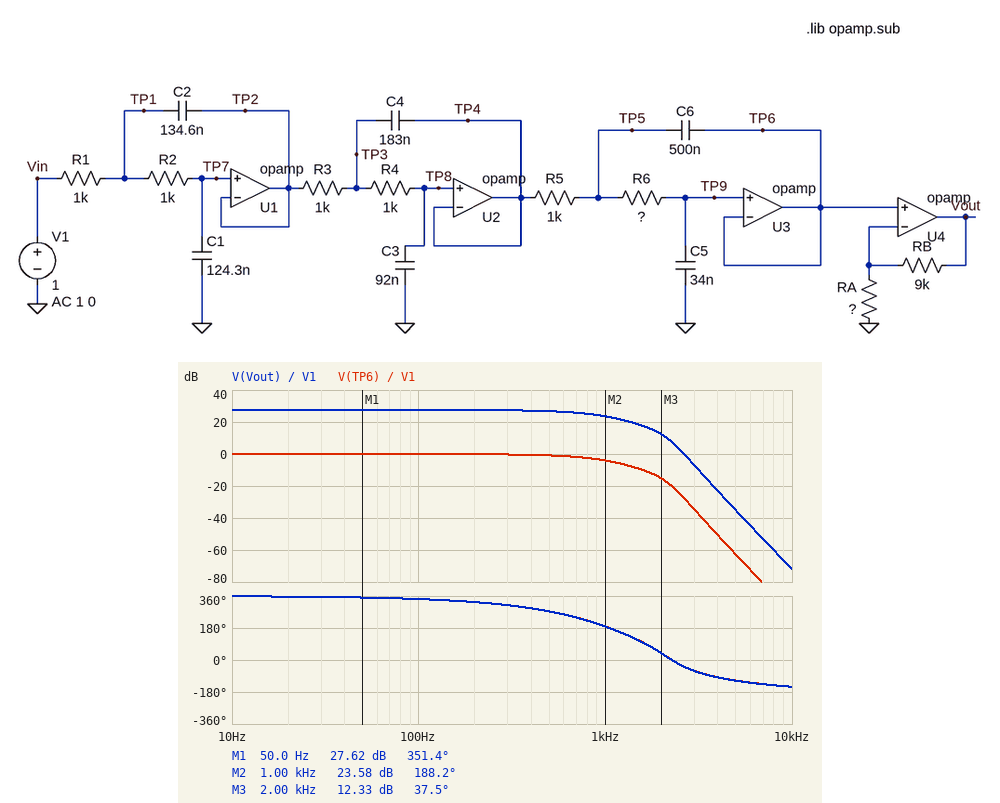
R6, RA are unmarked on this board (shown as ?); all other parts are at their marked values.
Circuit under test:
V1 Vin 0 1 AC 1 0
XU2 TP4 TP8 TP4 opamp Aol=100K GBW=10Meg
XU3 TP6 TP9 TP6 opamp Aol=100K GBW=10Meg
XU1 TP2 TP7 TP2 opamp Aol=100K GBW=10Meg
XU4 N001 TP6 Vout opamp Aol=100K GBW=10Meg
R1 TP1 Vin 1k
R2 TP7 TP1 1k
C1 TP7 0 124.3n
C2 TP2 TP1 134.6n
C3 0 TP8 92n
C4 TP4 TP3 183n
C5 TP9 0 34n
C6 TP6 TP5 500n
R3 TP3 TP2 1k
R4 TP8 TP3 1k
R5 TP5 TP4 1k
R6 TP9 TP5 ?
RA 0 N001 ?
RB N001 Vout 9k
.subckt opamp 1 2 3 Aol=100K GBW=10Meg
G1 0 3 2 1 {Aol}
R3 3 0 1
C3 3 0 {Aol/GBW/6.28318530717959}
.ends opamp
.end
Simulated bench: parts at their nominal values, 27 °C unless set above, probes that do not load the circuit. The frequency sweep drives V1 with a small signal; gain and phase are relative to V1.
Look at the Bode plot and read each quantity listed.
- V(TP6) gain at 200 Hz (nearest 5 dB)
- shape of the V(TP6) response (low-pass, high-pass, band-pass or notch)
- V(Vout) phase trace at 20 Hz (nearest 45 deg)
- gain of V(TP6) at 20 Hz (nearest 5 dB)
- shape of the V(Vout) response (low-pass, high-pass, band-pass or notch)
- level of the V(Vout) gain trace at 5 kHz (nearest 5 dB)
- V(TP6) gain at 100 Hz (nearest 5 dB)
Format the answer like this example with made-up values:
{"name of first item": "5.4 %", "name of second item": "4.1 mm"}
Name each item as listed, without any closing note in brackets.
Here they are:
{"V(TP6) gain at 200 Hz": "0 dB", "shape of the V(TP6) response": "low-pass", "V(Vout) phase trace at 20 Hz": "360 deg", "gain of V(TP6) at 20 Hz": "0 dB", "shape of the V(Vout) response": "low-pass", "level of the V(Vout) gain trace at 5 kHz": "-35 dB", "V(TP6) gain at 100 Hz": "0 dB"}
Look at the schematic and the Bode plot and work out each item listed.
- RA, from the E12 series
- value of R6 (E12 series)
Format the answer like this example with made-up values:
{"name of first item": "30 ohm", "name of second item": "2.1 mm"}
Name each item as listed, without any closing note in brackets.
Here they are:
{"RA, from the E12 series": "390 Ω", "value of R6": "330 Ω"}
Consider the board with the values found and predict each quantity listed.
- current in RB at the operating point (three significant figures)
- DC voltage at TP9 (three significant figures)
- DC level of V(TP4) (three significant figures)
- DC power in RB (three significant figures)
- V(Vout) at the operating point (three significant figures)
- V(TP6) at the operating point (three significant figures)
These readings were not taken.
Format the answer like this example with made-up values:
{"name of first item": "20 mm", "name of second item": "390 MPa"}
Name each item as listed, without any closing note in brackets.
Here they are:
{"current in RB at the operating point": "2.56 mA", "DC voltage at TP9": "1.00 V", "DC level of V(TP4)": "1.00 V", "DC power in RB": "59.1 mW", "V(Vout) at the operating point": "24.1 V", "V(TP6) at the operating point": "1.00 V"}
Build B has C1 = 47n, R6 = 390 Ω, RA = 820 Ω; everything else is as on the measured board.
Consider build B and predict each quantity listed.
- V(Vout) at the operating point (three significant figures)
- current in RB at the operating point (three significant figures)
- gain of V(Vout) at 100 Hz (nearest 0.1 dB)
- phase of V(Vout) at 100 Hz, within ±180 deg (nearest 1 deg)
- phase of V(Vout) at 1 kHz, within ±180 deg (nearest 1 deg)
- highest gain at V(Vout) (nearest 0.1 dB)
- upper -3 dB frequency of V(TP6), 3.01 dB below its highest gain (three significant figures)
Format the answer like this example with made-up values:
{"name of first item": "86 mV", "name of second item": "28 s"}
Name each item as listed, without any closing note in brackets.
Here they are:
{"V(Vout) at the operating point": "12.0 V", "current in RB at the operating point": "1.22 mA", "gain of V(Vout) at 100 Hz": "21.6 dB", "phase of V(Vout) at 100 Hz, within ±180 deg": "-12 deg", "phase of V(Vout) at 1 kHz, within ±180 deg": "-134 deg", "highest gain at V(Vout)": "22.4 dB", "upper -3 dB frequency of V(TP6), 3.01 dB below its highest gain": "1.71 kHz"}
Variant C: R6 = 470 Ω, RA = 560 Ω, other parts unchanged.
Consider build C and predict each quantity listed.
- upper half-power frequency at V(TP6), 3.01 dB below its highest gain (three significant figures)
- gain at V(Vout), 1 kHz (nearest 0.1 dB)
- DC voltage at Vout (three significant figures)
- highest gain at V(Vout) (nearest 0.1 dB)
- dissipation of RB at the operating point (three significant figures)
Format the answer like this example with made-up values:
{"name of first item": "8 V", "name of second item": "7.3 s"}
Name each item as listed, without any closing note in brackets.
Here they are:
{"upper half-power frequency at V(TP6), 3.01 dB below its highest gain": "970 Hz", "gain at V(Vout), 1 kHz": "21.4 dB", "DC voltage at Vout": "17.1 V", "highest gain at V(Vout)": "24.6 dB", "dissipation of RB at the operating point": "28.7 mW"}
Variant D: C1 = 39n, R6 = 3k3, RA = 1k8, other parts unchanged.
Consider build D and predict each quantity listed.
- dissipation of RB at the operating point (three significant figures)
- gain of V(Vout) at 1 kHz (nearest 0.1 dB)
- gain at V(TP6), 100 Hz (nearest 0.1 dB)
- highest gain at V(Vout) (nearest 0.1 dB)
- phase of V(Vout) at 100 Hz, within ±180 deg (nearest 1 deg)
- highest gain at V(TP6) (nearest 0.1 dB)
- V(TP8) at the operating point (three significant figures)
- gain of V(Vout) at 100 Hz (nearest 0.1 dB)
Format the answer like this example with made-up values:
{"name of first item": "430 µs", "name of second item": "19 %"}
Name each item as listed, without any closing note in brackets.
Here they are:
{"dissipation of RB at the operating point": "2.78 mW", "gain of V(Vout) at 1 kHz": "10.9 dB", "gain at V(TP6), 100 Hz": "0.2 dB", "highest gain at V(Vout)": "20.2 dB", "phase of V(Vout) at 100 Hz, within ±180 deg": "-15 deg", "highest gain at V(TP6)": "4.6 dB", "V(TP8) at the operating point": "1.00 V", "gain of V(Vout) at 100 Hz": "15.7 dB"}
